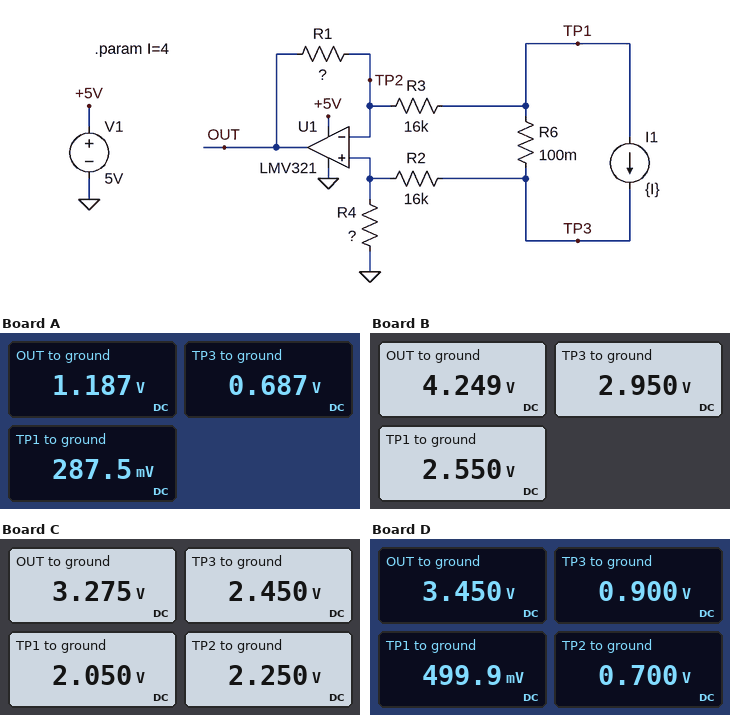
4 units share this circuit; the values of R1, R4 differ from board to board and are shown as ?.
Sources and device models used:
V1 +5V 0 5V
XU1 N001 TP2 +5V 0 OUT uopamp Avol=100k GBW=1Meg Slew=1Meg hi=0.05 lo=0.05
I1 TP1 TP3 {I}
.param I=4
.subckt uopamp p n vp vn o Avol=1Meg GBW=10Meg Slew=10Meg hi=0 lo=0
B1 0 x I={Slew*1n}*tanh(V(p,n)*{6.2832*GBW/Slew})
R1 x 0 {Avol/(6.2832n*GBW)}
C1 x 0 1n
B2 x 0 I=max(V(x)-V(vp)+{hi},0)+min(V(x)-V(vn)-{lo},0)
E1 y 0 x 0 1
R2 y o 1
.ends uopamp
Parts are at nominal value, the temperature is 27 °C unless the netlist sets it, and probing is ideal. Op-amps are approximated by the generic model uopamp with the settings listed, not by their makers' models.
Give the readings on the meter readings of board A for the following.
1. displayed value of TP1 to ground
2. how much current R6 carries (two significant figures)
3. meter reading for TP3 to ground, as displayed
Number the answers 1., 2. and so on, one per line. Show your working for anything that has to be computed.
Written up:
1. 287.5 mV
2. (687 mV - 287.5 mV) / 100 mΩ = 4.0 A
3. 0.687 V
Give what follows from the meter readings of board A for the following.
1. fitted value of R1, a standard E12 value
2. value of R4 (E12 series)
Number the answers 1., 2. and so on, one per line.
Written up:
1. 56 kΩ
2. 39 kΩ
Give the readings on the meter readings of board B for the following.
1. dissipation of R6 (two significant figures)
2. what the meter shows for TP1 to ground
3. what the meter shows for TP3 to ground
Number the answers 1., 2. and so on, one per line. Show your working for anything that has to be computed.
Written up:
1. (2.95 V - 2.55 V)^2 / 100 mΩ = 1.6 W
2. 2.550 V
3. 2.950 V
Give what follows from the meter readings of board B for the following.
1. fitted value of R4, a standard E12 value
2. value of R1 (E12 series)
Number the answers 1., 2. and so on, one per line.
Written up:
1. 220 kΩ
2. 120 kΩ
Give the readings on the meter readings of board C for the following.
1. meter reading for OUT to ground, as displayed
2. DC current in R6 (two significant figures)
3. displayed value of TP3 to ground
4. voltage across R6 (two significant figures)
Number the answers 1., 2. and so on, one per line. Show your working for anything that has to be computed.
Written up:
1. 3.275 V
2. (2.45 V - 2.05 V) / 100 mΩ = 4.0 A
3. 2.450 V
4. 2.45 V - 2.05 V = 400 mV
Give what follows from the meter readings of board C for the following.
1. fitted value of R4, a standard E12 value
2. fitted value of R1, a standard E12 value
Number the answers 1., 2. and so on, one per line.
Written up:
1. 180 kΩ
2. 82 kΩ
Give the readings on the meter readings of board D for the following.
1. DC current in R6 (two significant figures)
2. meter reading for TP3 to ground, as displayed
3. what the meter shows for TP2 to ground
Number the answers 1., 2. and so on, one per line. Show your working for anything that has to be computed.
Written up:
1. (900 mV - 499.9 mV) / 100 mΩ = 4.0 A
2. 0.900 V
3. 0.700 V
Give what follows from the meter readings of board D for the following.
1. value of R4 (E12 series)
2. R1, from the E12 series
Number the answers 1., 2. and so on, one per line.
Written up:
1. 56 kΩ
2. 220 kΩ
